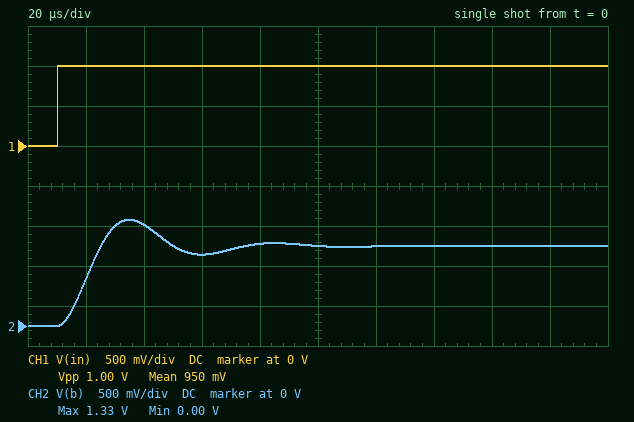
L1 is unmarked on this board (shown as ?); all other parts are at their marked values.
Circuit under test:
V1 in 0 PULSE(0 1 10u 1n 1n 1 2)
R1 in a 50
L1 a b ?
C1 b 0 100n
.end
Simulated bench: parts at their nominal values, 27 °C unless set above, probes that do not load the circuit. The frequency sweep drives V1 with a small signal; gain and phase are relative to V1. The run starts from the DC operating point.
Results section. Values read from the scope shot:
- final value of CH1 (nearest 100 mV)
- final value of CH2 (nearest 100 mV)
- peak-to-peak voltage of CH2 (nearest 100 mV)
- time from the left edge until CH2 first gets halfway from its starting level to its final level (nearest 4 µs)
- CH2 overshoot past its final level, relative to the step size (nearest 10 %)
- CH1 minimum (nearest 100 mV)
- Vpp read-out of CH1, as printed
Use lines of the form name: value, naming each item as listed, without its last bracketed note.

final value of CH1: 1.0 V
final value of CH2: 1.0 V
peak-to-peak voltage of CH2: 1.3 V
time from the left edge until CH2 first gets halfway from its starting level to its final level: 20 µs
CH2 overshoot past its final level, relative to the step size: 30 %
CH1 minimum: 0 V
Vpp read-out of CH1, as printed: 1.00 V
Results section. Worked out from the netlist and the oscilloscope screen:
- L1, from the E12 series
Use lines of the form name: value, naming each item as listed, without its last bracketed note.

L1, from the E12 series: 560 µH
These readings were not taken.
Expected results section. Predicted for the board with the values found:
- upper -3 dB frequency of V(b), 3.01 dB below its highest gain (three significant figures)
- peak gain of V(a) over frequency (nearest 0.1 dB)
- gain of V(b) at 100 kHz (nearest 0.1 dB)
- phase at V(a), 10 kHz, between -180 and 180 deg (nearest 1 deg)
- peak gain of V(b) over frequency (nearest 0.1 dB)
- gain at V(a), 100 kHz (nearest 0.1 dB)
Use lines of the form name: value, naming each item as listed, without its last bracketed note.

upper -3 dB frequency of V(b), 3.01 dB below its highest gain: 25.2 kHz
peak gain of V(a) over frequency: 0 dB
gain of V(b) at 100 kHz: -26.6 dB
phase at V(a), 10 kHz, between -180 and 180 deg: -22 deg
peak gain of V(b) over frequency: 4.0 dB
gain at V(a), 100 kHz: -0.1 dB
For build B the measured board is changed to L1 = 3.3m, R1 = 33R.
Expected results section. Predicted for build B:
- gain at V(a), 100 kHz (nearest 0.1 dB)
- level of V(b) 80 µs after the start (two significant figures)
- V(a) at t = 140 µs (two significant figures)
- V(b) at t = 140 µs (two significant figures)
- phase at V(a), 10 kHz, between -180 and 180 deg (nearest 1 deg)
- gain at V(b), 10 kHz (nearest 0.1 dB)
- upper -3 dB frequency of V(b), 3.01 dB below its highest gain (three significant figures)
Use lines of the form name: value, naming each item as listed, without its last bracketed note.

gain at V(a), 100 kHz: 0 dB
level of V(b) 80 µs after the start: 1.6 V
V(a) at t = 140 µs: 930 mV
V(b) at t = 140 µs: 620 mV
phase at V(a), 10 kHz, between -180 and 180 deg: 34 deg
gain at V(b), 10 kHz: 8.7 dB
upper -3 dB frequency of V(b), 3.01 dB below its highest gain: 9.45 kHz
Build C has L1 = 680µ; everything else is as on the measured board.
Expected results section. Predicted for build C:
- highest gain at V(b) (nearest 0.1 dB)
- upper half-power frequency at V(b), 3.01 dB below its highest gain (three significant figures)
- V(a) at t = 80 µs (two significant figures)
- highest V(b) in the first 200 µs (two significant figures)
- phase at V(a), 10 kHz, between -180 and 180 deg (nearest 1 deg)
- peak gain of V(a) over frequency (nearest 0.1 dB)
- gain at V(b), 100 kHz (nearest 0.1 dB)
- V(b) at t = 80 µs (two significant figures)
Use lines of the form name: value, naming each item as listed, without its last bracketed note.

highest gain at V(b): 4.8 dB
upper half-power frequency at V(b), 3.01 dB below its highest gain: 22.8 kHz
V(a) at t = 80 µs: 950 mV
highest V(b) in the first 200 µs: 1.4 V
phase at V(a), 10 kHz, between -180 and 180 deg: -23 deg
peak gain of V(a) over frequency: 0 dB
gain at V(b), 100 kHz: -28.3 dB
V(b) at t = 80 µs: 990 mV
